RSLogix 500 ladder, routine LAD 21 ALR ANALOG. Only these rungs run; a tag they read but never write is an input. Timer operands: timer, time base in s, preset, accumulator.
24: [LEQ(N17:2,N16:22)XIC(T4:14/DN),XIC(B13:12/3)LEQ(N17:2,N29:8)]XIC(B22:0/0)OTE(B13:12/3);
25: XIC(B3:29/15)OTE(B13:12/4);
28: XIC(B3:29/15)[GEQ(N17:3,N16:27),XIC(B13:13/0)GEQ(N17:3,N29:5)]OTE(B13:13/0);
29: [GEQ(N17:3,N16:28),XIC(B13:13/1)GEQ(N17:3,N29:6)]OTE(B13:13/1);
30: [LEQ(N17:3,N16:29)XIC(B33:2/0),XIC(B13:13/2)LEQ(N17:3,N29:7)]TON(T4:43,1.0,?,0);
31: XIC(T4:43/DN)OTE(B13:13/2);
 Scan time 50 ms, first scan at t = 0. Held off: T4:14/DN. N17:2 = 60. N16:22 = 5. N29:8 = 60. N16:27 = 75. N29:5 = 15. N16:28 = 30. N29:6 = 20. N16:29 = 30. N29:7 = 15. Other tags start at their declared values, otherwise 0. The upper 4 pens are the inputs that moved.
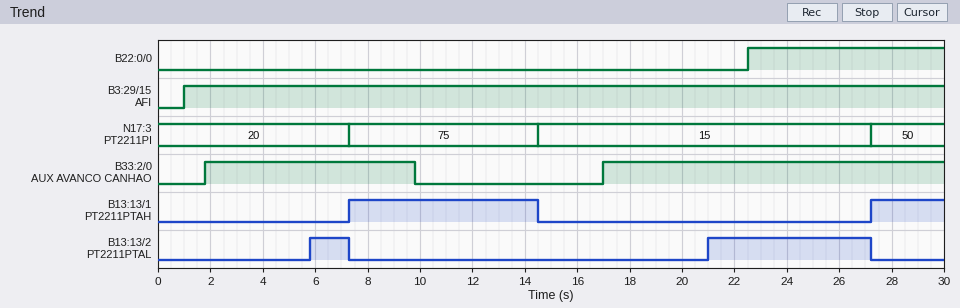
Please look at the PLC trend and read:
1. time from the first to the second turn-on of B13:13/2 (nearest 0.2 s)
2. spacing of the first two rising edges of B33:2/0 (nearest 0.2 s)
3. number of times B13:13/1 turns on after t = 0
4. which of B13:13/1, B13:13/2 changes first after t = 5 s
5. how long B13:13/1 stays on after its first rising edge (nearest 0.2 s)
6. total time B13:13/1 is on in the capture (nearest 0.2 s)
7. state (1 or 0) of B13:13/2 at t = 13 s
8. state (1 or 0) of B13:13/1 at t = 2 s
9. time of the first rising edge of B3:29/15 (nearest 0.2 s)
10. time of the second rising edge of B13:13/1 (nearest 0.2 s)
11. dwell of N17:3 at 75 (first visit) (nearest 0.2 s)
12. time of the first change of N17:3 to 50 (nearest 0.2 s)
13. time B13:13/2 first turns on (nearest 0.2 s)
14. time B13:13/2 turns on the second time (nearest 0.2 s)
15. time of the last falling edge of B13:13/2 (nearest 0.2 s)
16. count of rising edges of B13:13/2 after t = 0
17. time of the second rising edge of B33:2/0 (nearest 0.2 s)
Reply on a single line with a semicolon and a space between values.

15.2 s; 15.2 s; 2; B13:13/2; 7.2 s; 10.0 s; 0; 0; 1.0 s; 27.2 s; 7.2 s; 27.2 s; 5.8 s; 21.0 s; 27.2 s; 2; 17.0 s
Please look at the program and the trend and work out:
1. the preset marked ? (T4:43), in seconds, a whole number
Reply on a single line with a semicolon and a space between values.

4 s
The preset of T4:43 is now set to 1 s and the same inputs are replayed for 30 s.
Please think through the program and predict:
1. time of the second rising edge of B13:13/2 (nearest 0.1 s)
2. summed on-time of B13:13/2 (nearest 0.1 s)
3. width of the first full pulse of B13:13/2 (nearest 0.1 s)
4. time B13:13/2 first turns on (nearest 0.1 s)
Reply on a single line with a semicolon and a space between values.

18.0 s; 13.7 s; 4.5 s; 2.8 s
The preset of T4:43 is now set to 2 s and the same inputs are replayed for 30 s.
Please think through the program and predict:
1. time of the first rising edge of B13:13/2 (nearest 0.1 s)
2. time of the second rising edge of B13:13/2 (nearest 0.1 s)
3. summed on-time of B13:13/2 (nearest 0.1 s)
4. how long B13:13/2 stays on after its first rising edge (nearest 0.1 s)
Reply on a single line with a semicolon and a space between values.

3.8 s; 19.0 s; 11.7 s; 3.5 s
